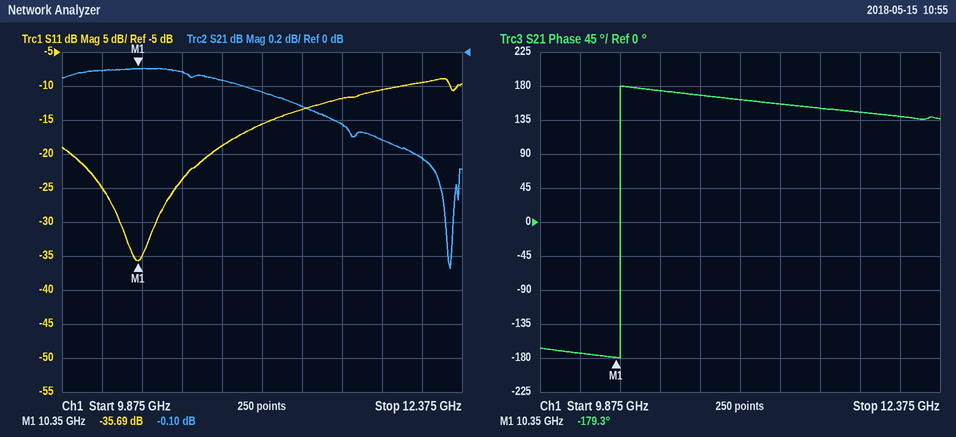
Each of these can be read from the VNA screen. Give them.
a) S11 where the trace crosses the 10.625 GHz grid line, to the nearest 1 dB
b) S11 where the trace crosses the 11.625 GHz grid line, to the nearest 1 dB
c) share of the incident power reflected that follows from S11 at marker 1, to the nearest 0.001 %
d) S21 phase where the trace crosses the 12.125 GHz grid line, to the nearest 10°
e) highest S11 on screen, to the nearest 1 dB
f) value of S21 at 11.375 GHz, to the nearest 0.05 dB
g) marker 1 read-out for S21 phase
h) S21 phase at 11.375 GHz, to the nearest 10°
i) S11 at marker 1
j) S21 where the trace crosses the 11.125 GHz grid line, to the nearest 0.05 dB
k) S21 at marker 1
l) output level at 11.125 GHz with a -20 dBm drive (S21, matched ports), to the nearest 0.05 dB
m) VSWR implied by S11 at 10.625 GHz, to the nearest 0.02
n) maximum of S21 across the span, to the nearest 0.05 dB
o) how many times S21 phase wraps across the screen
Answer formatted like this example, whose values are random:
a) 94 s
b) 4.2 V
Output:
a) -24 dB
b) -12 dB
c) 0.027 %
d) 140°
e) -9 dB
f) -0.30 dB
g) -179.3°
h) 160°
i) -35.69 dB
j) -0.25 dB
k) -0.10 dB
l) -20.25 dBm
m) 1.14
n) -0.10 dB
o) 1
